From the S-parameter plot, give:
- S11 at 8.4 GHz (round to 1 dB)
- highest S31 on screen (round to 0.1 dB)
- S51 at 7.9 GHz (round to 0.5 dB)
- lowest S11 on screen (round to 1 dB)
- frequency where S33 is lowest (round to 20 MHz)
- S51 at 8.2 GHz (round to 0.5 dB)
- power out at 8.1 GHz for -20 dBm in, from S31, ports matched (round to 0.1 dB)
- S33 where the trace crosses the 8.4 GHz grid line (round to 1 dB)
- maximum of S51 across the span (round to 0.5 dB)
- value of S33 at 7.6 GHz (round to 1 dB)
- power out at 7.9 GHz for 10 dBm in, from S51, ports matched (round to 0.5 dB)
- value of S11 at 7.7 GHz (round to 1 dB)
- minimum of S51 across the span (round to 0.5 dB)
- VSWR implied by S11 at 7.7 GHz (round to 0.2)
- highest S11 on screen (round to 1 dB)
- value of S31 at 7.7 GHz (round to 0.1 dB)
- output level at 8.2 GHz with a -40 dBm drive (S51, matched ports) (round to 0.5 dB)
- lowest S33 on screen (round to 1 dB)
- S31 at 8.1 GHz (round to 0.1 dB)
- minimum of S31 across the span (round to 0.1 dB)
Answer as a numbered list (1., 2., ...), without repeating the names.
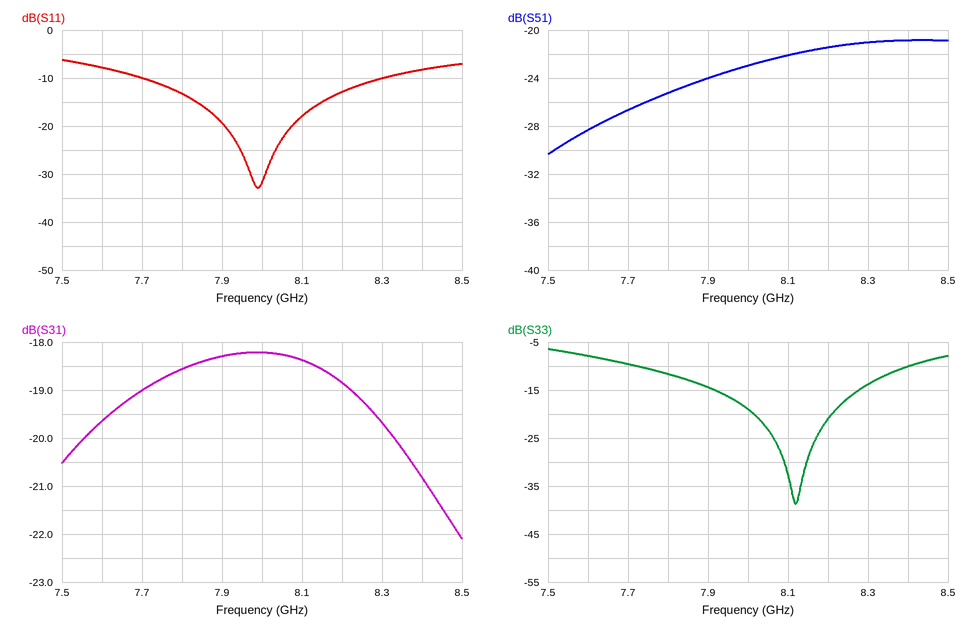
1. -8 dB
2. -18.2 dB
3. -24.0 dB
4. -33 dB
5. 8.12 GHz
6. -21.5 dB
7. -38.4 dBm
8. -10 dB
9. -21.0 dB
10. -8 dB
11. -14.0 dBm
12. -10 dB
13. -30.5 dB
14. 2.0
15. -6 dB
16. -19.0 dB
17. -61.5 dBm
18. -39 dB
19. -18.4 dB
20. -22.1 dB
